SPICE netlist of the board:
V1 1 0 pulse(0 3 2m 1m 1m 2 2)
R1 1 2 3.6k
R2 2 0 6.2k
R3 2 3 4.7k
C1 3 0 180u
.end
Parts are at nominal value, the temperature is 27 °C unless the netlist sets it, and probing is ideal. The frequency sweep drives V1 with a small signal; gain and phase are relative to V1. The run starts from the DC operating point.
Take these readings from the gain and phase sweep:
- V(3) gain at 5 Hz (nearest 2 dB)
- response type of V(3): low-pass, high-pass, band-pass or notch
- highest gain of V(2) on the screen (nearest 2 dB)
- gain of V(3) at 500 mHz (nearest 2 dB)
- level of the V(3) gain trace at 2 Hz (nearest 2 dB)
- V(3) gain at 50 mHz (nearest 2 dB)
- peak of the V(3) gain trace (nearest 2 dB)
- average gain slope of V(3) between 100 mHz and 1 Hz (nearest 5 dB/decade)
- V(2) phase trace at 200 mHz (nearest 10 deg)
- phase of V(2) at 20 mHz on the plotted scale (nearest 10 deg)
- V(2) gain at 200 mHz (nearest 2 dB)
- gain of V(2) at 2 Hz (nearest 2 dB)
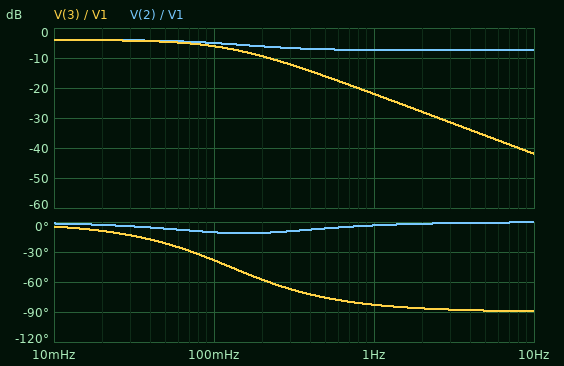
-36 dB
low-pass
-4 dB
-16 dB
-28 dB
-4 dB
-4 dB
-15 dB/decade
-10 deg
0 deg
-6 dB
-8 dB
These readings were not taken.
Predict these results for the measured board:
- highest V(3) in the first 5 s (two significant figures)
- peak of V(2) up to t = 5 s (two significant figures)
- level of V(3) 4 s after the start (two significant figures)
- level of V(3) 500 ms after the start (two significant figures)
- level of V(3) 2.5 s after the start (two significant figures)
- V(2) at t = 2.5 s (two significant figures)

1.9 V
1.9 V
1.8 V
620 mV
1.6 V
1.8 V
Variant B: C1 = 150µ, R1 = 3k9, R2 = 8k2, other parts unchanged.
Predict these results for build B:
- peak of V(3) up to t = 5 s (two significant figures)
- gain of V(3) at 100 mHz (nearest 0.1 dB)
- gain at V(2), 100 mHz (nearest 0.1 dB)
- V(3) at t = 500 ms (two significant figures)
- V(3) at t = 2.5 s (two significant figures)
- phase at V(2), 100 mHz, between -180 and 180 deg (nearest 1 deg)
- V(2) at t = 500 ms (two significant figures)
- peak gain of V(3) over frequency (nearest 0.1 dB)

2.0 V
-5.1 dB
-4.3 dB
740 mV
1.8 V
-11 deg
1.6 V
-3.4 dB
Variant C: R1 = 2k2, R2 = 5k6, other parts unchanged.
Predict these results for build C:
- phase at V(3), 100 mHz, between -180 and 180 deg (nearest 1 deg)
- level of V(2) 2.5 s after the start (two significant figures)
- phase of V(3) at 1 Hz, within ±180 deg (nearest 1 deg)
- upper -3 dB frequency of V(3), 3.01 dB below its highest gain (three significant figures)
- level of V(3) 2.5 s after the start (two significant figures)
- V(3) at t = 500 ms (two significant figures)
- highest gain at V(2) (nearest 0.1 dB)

-35 deg
2.1 V
-82 deg
141 mHz
1.9 V
770 mV
-2.9 dB
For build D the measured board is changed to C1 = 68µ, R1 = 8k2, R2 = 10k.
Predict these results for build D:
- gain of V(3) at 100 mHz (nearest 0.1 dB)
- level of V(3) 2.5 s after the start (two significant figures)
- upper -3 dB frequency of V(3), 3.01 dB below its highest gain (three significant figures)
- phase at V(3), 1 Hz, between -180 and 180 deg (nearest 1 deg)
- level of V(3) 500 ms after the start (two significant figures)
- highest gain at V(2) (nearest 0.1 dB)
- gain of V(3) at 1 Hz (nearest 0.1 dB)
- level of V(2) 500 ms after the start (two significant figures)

-5.8 dB
1.6 V
254 mHz
-76 deg
900 mV
-5.2 dB
-17.4 dB
1.3 V
